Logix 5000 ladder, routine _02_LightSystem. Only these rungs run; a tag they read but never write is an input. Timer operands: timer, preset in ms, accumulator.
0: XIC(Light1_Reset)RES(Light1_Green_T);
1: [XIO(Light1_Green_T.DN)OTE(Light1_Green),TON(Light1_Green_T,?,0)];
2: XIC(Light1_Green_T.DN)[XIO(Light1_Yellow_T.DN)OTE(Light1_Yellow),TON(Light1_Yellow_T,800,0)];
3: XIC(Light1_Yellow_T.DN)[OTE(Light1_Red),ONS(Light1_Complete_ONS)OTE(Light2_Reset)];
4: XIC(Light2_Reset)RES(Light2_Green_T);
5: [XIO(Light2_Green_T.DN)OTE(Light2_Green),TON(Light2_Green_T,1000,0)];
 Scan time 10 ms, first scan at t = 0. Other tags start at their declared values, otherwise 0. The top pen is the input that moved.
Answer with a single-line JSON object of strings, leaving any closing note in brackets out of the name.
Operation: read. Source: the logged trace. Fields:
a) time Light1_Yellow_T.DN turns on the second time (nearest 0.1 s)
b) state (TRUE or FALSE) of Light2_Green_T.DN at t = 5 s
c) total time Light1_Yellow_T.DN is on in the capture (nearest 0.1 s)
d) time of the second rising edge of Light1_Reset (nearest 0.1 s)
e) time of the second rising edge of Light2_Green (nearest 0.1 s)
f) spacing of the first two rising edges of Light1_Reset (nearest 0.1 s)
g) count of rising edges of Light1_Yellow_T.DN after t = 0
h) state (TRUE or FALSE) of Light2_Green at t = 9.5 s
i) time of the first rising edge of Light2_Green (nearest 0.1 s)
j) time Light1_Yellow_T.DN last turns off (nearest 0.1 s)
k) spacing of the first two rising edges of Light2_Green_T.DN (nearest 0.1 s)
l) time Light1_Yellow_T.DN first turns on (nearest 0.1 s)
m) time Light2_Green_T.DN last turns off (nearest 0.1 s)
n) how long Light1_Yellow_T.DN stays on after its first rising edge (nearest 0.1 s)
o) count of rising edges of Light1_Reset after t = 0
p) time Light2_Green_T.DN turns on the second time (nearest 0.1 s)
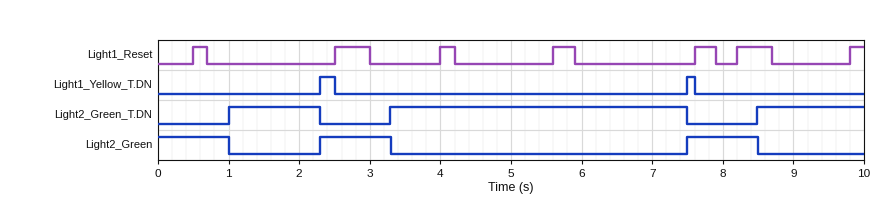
{"time Light1_Yellow_T.DN turns on the second time": "7.5 s", "state (TRUE or FALSE) of Light2_Green_T.DN at t = 5 s": "TRUE", "total time Light1_Yellow_T.DN is on in the capture": "0.3 s", "time of the second rising edge of Light1_Reset": "2.5 s", "time of the second rising edge of Light2_Green": "7.5 s", "spacing of the first two rising edges of Light1_Reset": "2.0 s", "count of rising edges of Light1_Yellow_T.DN after t = 0": "2", "state (TRUE or FALSE) of Light2_Green at t = 9.5 s": "FALSE", "time of the first rising edge of Light2_Green": "2.3 s", "time Light1_Yellow_T.DN last turns off": "7.6 s", "spacing of the first two rising edges of Light2_Green_T.DN": "2.3 s", "time Light1_Yellow_T.DN first turns on": "2.3 s", "time Light2_Green_T.DN last turns off": "7.5 s", "how long Light1_Yellow_T.DN stays on after its first rising edge": "0.2 s", "count of rising edges of Light1_Reset after t = 0": "7", "time Light2_Green_T.DN turns on the second time": "3.3 s"}
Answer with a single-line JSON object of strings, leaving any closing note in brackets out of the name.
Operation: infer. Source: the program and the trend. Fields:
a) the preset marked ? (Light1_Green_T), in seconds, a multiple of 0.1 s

{"the preset marked ? (Light1_Green_T), in seconds, a multiple of 0.1 s": "0.8 s"}
